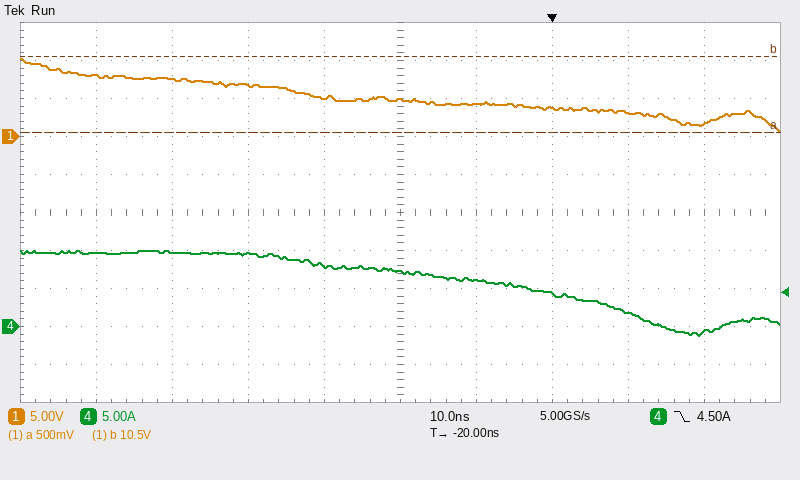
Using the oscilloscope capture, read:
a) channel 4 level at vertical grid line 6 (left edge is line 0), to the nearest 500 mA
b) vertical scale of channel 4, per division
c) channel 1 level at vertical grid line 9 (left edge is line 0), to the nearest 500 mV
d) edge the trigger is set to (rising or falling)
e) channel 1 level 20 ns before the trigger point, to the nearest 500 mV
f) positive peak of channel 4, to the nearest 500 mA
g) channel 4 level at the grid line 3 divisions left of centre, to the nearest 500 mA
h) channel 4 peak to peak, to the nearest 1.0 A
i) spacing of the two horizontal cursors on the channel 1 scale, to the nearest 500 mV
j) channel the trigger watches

6.0 A
5 A
1.5 V
falling
5.0 V
10.0 A
10.0 A
11.0 A
10.0 V
channel 4
